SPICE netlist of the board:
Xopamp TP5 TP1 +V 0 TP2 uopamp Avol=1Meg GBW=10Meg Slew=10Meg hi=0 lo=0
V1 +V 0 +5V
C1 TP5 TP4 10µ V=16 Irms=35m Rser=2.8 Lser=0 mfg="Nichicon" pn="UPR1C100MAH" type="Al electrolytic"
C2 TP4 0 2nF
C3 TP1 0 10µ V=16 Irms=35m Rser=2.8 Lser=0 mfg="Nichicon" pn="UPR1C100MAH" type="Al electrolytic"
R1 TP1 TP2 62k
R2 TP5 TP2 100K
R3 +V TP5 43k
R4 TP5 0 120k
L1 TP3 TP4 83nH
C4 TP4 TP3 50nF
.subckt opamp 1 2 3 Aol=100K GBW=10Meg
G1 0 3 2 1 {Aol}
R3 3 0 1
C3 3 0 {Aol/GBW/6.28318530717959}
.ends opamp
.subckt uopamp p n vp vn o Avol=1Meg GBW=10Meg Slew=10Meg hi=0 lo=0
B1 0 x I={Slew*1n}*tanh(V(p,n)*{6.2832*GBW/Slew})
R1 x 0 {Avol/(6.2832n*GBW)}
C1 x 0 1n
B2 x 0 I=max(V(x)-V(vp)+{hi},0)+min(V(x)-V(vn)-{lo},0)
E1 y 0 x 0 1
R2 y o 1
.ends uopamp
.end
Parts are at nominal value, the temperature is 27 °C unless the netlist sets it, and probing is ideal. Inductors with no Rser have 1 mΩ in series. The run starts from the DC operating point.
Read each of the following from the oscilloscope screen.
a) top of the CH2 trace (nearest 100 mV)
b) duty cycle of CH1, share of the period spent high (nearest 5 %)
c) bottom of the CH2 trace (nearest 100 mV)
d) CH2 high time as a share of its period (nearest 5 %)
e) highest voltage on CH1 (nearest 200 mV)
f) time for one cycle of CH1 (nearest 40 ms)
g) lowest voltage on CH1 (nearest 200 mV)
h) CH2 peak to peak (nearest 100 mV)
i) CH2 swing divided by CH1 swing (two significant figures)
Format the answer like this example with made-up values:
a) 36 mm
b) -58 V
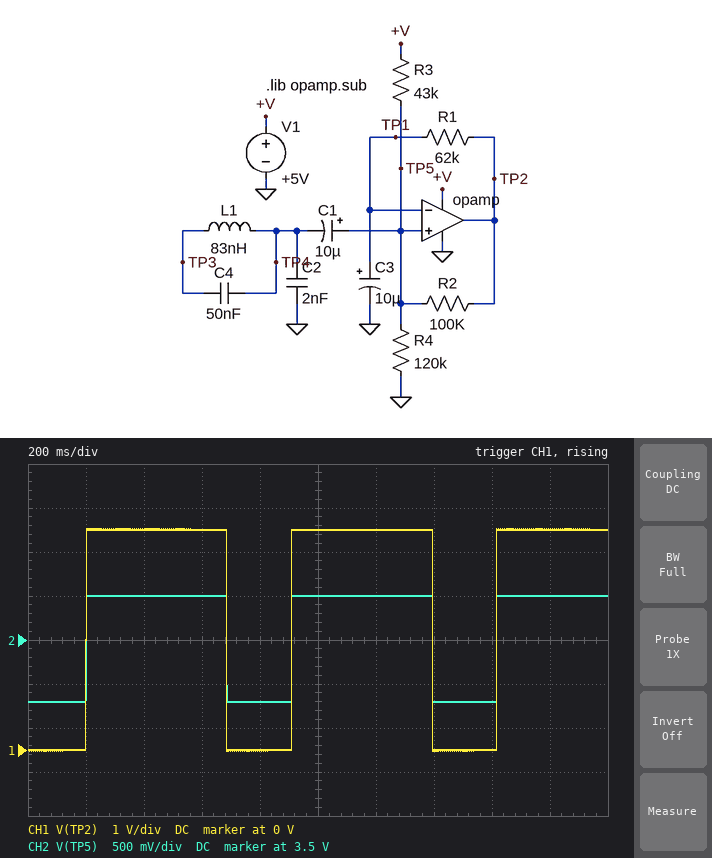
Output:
a) 4.0 V
b) 70 %
c) 2.8 V
d) 70 %
e) 5.0 V
f) 720 ms
g) 0 V
h) 1.2 V
i) 0.24
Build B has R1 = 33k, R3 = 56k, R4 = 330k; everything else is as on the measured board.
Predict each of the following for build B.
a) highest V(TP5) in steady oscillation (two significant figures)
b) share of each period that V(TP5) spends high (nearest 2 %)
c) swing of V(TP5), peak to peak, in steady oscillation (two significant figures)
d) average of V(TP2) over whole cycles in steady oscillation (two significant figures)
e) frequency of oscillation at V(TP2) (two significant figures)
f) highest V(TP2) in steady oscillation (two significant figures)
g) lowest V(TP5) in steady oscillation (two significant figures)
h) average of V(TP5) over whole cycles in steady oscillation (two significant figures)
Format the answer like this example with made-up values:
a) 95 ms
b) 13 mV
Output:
a) 4.5 V
b) 76 %
c) 1.6 V
d) 3.8 V
e) 1.6 Hz
f) 5.0 V
g) 2.9 V
h) 4.1 V
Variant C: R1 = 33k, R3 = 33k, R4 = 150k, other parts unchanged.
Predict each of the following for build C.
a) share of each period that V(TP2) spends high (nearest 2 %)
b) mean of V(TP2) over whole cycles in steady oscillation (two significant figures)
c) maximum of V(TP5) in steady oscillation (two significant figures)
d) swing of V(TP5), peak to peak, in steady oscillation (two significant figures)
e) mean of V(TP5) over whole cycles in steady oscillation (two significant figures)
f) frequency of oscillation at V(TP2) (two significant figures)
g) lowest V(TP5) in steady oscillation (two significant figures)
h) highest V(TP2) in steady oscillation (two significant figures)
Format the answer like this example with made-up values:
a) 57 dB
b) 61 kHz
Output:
a) 76 %
b) 3.8 V
c) 4.3 V
d) 1.1 V
e) 4.0 V
f) 2.5 Hz
g) 3.2 V
h) 5.0 V
